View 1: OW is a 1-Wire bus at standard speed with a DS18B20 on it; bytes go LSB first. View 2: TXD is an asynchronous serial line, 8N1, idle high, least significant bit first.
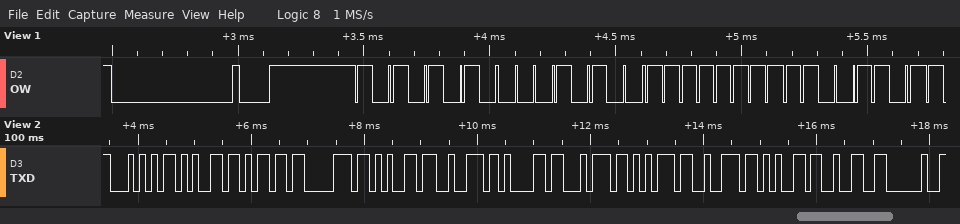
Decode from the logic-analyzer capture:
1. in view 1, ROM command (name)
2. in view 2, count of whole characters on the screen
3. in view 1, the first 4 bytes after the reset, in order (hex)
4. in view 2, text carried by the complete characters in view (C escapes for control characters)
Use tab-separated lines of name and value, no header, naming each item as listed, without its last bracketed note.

in view 1, ROM command	Match ROM
in view 2, count of whole characters on the screen	13
in view 1, the first 4 bytes after the reset, in order	55 28 FF B3
in view 2, text carried by the complete characters in view	"Temperature2 "
